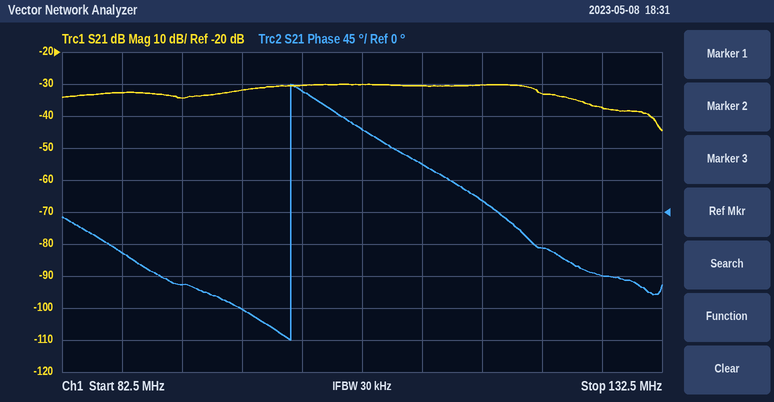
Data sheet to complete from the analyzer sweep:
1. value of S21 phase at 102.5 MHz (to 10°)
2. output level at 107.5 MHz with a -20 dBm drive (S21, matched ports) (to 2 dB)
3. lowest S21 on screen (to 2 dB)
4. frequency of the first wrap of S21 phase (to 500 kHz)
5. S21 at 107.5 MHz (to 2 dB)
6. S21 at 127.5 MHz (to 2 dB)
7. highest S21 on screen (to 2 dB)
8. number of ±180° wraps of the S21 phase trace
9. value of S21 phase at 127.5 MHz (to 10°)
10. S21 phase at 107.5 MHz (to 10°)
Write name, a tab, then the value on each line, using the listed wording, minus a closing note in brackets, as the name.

value of S21 phase at 102.5 MHz	170°
output level at 107.5 MHz with a -20 dBm drive (S21, matched ports)	-50 dBm
lowest S21 on screen	-44 dB
frequency of the first wrap of S21 phase	101.5 MHz
S21 at 107.5 MHz	-30 dB
S21 at 127.5 MHz	-38 dB
highest S21 on screen	-30 dB
number of ±180° wraps of the S21 phase trace	1
value of S21 phase at 127.5 MHz	-90°
S21 phase at 107.5 MHz	120°
